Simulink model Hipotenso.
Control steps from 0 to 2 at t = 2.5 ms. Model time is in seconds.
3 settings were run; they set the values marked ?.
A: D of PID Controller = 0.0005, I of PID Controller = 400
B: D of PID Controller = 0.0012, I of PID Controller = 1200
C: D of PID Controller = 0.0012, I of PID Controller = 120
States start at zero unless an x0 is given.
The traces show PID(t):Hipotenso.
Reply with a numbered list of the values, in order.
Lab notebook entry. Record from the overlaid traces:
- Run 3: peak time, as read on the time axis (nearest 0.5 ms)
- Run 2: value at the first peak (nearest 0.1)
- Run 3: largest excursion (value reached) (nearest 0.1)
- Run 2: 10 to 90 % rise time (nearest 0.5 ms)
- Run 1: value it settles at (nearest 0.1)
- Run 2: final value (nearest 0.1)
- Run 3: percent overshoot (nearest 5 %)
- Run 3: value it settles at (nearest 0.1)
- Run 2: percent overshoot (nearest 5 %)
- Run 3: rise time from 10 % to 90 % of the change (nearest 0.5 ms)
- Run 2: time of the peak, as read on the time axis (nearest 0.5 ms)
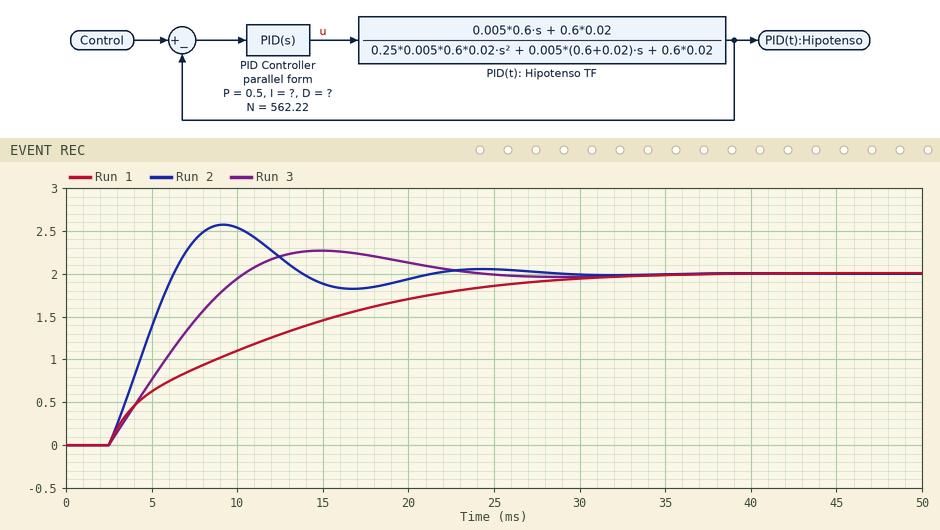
1. 15.0 ms
2. 2.6
3. 2.3
4. 3.0 ms
5. 2.0
6. 2.0
7. 15 %
8. 2.0
9. 30 %
10. 6.0 ms
11. 9.0 ms
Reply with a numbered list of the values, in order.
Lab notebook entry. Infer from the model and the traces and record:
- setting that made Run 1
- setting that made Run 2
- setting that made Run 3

1. C
2. B
3. A
